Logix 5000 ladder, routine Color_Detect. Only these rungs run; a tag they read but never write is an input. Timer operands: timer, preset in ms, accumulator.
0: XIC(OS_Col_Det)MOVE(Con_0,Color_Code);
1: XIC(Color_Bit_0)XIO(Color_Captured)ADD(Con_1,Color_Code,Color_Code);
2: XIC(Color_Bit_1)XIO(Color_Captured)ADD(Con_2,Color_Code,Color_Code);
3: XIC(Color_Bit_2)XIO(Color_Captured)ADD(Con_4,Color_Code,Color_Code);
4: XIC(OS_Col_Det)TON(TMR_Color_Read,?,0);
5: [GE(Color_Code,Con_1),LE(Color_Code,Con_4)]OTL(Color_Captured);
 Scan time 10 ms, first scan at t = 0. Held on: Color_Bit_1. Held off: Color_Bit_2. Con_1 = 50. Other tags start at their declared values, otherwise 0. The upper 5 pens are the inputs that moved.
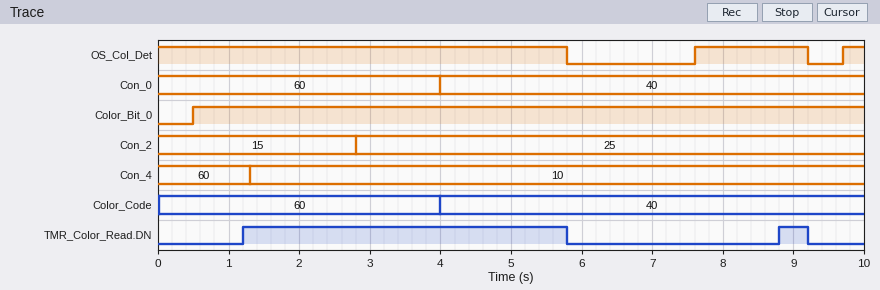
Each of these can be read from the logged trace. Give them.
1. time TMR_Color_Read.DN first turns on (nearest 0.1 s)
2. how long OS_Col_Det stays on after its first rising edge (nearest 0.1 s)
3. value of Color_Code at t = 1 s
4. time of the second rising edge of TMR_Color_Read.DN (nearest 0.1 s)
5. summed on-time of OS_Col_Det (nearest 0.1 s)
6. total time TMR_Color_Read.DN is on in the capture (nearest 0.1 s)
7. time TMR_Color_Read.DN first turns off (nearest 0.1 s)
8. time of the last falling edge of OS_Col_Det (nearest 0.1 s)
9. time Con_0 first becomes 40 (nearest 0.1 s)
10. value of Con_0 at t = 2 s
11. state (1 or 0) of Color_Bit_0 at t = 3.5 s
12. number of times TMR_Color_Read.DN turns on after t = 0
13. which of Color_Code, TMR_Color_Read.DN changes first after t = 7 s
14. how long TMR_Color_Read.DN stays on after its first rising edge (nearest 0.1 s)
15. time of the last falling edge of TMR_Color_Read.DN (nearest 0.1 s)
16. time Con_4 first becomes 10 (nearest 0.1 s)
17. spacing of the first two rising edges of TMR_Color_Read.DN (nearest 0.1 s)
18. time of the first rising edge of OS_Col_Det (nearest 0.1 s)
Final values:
1.2 s
1.6 s
60
8.8 s
7.7 s
5.0 s
5.8 s
9.2 s
4.0 s
60
1
2
TMR_Color_Read.DN
4.6 s
9.2 s
1.3 s
7.6 s
7.6 s
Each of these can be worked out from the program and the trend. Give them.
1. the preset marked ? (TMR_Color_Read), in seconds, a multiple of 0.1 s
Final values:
1.2 s
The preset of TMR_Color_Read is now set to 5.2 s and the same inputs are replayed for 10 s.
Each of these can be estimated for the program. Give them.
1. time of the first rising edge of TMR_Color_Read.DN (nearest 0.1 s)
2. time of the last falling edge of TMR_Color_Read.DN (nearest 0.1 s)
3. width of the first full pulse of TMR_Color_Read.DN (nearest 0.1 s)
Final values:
5.2 s
5.8 s
0.6 s
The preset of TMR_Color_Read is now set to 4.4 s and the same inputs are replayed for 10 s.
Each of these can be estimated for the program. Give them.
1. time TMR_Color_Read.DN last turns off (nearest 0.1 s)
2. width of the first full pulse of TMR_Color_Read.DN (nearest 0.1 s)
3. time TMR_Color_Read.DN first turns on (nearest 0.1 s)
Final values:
5.8 s
1.4 s
4.4 s
